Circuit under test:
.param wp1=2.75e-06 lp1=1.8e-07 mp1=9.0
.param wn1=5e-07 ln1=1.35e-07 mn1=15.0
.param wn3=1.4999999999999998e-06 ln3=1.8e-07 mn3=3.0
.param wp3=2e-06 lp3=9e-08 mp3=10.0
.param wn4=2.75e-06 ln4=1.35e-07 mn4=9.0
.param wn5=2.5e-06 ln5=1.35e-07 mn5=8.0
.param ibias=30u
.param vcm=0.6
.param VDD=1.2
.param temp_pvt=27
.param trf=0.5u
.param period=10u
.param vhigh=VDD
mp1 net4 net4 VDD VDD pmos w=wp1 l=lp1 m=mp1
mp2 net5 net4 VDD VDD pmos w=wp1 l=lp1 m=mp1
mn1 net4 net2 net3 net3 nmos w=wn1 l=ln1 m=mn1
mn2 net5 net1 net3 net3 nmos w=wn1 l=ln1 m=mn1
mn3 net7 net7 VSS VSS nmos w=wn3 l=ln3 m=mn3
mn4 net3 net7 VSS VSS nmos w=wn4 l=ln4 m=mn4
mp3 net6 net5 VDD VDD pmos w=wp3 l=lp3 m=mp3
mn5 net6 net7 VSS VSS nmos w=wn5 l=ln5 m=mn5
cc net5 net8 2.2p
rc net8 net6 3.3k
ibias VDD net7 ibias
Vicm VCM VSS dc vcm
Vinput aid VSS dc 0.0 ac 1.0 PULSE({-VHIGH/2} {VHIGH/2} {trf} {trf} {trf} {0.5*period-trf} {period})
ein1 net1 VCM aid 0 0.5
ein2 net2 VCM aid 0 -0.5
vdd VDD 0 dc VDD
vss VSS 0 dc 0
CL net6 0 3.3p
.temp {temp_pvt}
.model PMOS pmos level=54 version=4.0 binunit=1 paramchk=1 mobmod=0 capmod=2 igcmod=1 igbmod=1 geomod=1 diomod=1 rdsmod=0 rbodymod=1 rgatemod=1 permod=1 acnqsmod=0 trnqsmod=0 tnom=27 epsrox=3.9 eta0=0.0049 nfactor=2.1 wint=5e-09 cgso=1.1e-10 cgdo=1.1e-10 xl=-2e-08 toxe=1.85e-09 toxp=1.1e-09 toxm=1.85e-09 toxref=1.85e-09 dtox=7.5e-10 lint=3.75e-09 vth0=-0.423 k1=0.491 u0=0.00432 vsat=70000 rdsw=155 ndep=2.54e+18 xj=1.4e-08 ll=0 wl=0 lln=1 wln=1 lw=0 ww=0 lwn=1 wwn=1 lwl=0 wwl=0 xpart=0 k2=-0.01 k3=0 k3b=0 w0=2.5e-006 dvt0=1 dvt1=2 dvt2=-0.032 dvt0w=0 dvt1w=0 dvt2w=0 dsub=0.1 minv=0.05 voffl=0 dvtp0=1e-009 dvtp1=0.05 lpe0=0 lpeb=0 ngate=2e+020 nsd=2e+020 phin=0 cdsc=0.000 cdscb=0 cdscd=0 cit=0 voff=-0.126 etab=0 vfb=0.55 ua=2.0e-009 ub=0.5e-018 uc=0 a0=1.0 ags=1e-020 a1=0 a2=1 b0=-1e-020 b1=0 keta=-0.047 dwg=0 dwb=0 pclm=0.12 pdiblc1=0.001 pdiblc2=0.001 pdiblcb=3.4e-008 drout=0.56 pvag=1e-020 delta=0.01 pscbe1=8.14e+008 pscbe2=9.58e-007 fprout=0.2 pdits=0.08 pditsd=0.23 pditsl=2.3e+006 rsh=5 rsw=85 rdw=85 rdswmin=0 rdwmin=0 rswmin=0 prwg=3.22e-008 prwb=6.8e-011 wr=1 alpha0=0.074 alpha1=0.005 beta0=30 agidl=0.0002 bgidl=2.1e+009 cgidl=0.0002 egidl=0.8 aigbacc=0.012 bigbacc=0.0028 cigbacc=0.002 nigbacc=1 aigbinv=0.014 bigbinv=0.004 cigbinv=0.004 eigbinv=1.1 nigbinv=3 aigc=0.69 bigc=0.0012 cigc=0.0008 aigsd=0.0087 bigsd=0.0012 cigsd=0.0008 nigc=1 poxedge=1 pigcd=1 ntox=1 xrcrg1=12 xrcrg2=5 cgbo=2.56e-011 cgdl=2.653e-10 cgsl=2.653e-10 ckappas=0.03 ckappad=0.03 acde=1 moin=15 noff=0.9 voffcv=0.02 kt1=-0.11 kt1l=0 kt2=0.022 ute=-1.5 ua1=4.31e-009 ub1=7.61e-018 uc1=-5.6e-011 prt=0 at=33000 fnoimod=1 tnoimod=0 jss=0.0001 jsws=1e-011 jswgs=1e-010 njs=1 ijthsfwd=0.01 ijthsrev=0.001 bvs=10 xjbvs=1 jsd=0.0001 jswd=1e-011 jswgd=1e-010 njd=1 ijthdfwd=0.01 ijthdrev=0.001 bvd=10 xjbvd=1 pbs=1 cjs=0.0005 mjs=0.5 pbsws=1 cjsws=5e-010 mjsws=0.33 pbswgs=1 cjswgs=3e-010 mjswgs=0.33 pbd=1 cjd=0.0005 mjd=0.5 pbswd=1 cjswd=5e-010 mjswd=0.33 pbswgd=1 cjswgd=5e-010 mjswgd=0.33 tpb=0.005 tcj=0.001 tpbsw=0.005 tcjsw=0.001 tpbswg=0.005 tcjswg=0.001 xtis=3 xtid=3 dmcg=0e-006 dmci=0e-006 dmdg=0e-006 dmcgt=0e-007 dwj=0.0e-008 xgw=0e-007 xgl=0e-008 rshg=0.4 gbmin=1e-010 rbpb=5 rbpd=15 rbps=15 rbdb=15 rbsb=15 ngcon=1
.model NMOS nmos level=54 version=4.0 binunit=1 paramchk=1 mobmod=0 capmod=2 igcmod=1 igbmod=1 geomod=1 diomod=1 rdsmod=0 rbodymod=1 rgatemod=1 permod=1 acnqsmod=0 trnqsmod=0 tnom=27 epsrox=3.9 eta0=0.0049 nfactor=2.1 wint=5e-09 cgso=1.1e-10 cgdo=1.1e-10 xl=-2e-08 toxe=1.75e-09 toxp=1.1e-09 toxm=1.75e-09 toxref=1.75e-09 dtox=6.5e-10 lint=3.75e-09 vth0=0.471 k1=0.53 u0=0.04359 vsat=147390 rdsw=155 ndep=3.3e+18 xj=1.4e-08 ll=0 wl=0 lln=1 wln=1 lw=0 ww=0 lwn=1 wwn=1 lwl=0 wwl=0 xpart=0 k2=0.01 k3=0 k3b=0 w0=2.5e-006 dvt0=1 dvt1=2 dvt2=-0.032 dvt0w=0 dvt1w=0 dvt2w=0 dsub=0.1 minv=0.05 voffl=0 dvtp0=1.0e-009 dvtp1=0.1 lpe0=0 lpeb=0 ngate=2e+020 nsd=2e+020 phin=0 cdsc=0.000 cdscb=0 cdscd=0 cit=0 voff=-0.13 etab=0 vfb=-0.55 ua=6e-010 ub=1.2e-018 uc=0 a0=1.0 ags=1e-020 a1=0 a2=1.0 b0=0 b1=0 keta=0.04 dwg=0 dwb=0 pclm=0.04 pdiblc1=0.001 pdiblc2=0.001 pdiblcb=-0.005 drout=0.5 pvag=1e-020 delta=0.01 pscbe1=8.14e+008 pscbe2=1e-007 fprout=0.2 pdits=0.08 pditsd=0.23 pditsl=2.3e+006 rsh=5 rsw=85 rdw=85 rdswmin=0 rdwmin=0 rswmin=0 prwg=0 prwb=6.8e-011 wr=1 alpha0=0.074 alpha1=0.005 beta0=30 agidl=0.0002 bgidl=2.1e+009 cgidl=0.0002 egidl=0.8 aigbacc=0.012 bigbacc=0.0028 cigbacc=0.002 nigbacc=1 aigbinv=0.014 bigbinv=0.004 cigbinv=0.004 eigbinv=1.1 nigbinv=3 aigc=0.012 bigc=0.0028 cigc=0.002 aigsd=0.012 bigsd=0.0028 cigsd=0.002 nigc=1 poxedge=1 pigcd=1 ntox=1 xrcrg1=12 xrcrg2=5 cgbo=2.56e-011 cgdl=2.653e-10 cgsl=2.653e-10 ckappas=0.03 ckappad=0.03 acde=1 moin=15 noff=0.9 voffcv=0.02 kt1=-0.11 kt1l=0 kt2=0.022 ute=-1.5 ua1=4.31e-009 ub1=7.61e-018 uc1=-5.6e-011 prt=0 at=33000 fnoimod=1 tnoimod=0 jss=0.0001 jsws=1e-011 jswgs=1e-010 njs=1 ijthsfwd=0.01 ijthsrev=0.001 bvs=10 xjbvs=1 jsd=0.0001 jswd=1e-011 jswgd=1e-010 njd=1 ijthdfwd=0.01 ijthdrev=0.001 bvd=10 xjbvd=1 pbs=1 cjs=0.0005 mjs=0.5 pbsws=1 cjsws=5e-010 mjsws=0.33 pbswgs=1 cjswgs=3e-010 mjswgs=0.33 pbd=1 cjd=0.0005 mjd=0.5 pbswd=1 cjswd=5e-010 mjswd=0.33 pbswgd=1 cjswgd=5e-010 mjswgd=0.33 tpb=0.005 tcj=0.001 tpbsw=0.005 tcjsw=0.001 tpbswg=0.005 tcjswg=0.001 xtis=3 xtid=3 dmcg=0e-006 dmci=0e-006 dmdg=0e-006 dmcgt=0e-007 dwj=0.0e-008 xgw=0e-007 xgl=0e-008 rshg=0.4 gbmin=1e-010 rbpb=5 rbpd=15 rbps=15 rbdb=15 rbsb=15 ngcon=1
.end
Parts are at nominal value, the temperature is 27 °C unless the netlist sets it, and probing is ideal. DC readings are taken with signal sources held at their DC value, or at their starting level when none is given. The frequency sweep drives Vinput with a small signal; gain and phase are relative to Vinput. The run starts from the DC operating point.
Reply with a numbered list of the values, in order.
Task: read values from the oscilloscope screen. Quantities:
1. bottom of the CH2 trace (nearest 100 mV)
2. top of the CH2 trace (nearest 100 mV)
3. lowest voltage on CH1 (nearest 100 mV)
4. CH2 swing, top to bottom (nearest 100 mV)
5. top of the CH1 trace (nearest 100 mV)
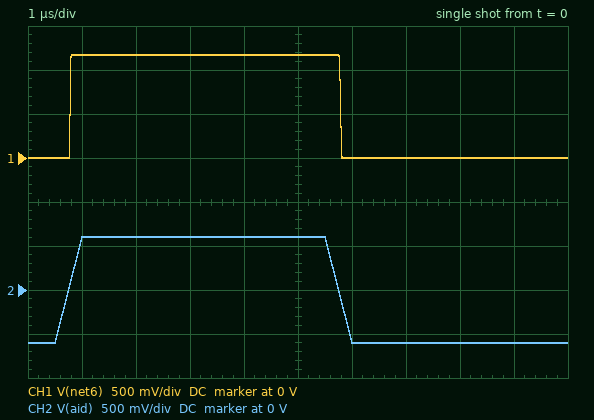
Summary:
1. -600 mV
2. 600 mV
3. 0 V
4. 1.2 V
5. 1.2 V
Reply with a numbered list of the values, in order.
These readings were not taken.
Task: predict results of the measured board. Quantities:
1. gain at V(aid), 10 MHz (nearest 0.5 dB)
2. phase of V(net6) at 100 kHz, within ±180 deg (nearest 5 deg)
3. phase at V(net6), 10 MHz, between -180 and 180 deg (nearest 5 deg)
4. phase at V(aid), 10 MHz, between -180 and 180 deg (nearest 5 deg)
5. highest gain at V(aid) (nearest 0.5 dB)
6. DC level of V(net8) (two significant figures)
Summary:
1. 0 dB
2. -35 deg
3. -75 deg
4. 0 deg
5. 0 dB
6. 990 mV
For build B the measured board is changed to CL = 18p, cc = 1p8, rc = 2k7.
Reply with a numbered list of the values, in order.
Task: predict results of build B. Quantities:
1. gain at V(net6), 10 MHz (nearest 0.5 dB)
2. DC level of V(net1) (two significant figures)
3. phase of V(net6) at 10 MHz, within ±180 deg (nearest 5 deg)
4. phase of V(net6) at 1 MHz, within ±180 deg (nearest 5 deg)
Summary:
1. 20.5 dB
2. 600 mV
3. -105 deg
4. -85 deg
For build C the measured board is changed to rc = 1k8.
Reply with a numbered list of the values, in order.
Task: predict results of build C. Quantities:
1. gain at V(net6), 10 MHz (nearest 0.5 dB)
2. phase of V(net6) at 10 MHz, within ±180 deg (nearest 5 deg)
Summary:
1. 20.5 dB
2. -85 deg
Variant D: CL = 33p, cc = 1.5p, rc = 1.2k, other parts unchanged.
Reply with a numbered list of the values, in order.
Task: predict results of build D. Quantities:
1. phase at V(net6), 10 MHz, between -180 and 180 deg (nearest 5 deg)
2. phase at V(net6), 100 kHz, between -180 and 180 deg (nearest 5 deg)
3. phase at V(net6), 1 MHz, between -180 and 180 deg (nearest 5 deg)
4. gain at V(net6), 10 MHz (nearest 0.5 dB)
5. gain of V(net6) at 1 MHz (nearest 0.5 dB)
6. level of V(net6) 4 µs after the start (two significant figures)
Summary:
1. -125 deg
2. -30 deg
3. -85 deg
4. 20.0 dB
5. 42.0 dB
6. 1.2 V
